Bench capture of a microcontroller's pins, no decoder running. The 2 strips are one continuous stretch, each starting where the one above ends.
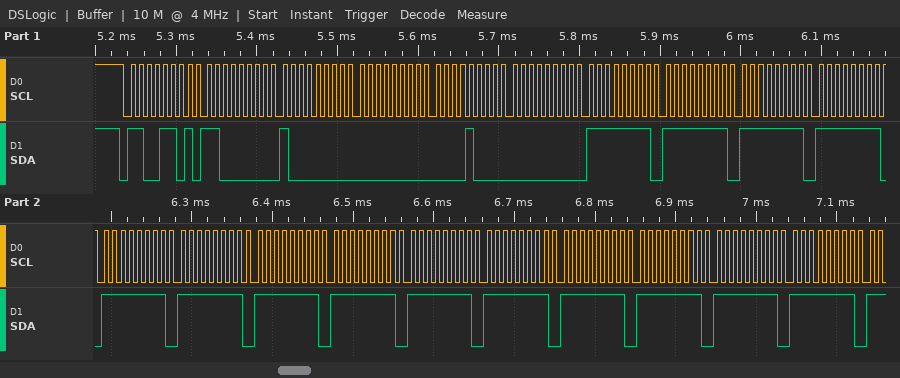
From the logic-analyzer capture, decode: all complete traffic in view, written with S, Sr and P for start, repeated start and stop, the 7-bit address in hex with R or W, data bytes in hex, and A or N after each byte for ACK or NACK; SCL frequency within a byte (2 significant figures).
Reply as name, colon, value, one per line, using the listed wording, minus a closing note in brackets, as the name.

all complete traffic in view, written with S, Sr and P for start, repeated start and stop, the 7-bit address in hex with R or W, data bytes in hex, and A or N after each byte for ACK or NACK: S 66R A C0 A 80 A 00 A 08 A 00 A FF A FF A FF A FF A FF A FF A FF A FF A FF A FF A FF A FF A FF A FF A
SCL frequency within a byte: 100 kHz
